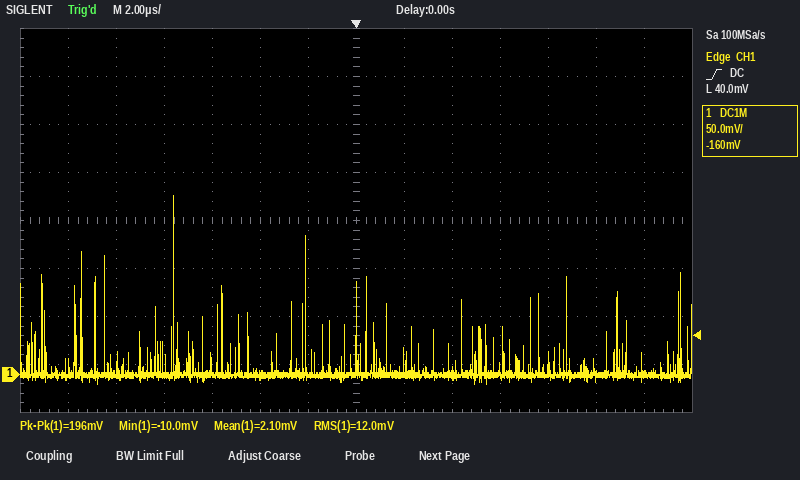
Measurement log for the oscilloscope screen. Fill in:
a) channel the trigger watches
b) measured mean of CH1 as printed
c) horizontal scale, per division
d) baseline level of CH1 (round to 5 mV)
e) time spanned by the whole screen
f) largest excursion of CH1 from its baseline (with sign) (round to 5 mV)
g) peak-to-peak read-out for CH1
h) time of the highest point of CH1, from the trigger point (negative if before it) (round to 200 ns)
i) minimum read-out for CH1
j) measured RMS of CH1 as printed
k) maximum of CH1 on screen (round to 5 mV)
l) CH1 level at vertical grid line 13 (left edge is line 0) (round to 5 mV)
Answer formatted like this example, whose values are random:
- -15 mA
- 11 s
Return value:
- CH1
- 2.10 mV
- 2 µs
- 0 mV
- 28 µs
- +185 mV
- 196 mV
- -7.6 µs
- -10.0 mV
- 12.0 mV
- 185 mV
- 0 mV
